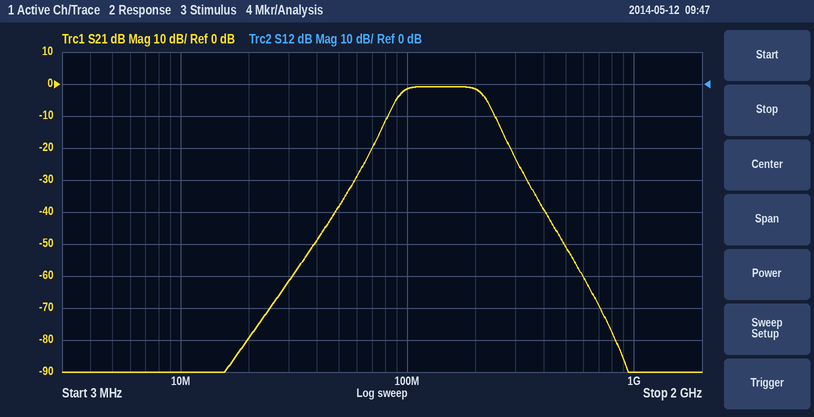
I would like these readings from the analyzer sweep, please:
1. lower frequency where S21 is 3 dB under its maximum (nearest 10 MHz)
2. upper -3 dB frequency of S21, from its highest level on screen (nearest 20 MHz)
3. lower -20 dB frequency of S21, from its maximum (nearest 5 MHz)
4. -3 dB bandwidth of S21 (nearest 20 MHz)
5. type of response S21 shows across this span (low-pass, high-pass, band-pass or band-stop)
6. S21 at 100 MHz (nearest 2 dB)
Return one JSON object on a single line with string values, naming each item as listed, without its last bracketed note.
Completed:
{"lower frequency where S21 is 3 dB under its maximum": "90 MHz", "upper -3 dB frequency of S21, from its highest level on screen": "220 MHz", "lower -20 dB frequency of S21, from its maximum": "70 MHz", "-3 dB bandwidth of S21": "120 MHz", "type of response S21 shows across this span": "band-pass", "S21 at 100 MHz": "-2 dB"}
